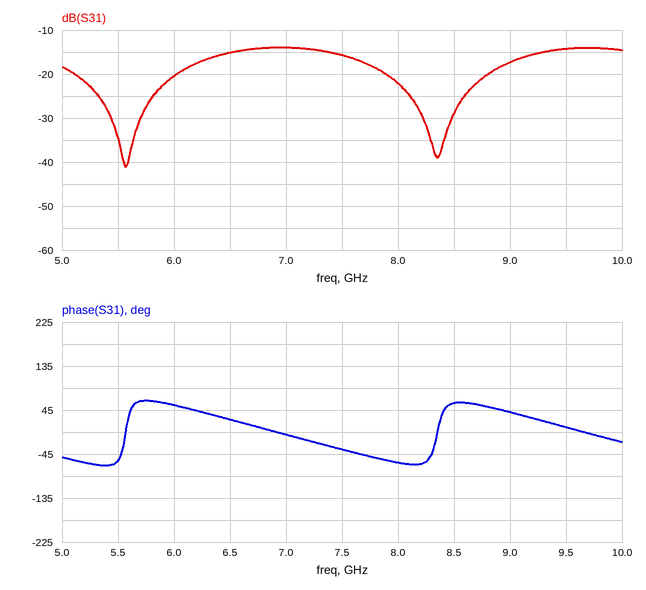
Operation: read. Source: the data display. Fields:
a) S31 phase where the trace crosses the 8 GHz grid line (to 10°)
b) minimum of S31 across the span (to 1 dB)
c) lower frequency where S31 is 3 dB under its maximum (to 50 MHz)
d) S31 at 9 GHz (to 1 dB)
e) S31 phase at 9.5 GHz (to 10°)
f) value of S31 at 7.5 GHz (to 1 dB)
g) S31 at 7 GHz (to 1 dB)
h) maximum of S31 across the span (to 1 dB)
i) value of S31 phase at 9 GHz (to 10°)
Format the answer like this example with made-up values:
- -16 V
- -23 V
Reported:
- -60°
- -41 dB
- 6.25 GHz
- -17 dB
- 10°
- -16 dB
- -14 dB
- -14 dB
- 40°
